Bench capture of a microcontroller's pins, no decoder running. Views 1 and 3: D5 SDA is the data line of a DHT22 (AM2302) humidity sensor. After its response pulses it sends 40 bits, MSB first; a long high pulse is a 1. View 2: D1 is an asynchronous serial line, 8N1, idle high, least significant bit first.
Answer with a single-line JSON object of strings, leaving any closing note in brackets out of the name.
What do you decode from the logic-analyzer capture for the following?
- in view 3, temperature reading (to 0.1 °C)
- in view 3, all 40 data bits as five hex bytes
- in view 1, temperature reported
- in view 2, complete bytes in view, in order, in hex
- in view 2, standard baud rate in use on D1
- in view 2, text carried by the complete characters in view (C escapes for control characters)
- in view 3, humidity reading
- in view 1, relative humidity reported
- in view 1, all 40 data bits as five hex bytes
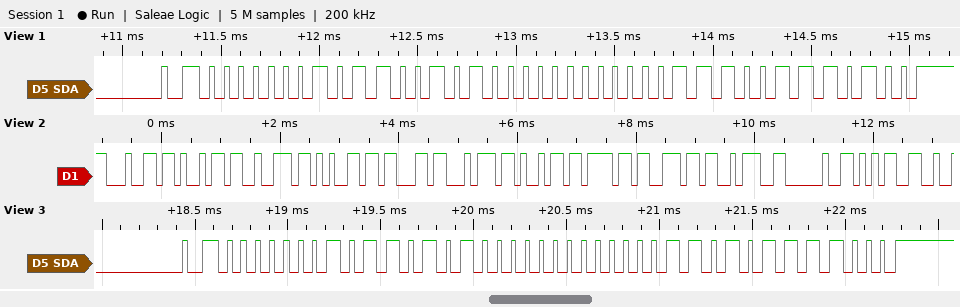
{"in view 3, temperature reading": "1.3 °C", "in view 3, all 40 data bits as five hex bytes": "01 6A 00 0D 78", "in view 1, temperature reported": "1.4 °C", "in view 2, complete bytes in view, in order, in hex": "64 69 72 65 63 74 69 6F 6E 3A 20 35", "in view 2, standard baud rate in use on D1": "9600 baud", "in view 2, text carried by the complete characters in view": "\"direction: 5\"", "in view 3, humidity reading": "36.2 %", "in view 1, relative humidity reported": "35.7 %", "in view 1, all 40 data bits as five hex bytes": "01 65 00 0E 74"}
